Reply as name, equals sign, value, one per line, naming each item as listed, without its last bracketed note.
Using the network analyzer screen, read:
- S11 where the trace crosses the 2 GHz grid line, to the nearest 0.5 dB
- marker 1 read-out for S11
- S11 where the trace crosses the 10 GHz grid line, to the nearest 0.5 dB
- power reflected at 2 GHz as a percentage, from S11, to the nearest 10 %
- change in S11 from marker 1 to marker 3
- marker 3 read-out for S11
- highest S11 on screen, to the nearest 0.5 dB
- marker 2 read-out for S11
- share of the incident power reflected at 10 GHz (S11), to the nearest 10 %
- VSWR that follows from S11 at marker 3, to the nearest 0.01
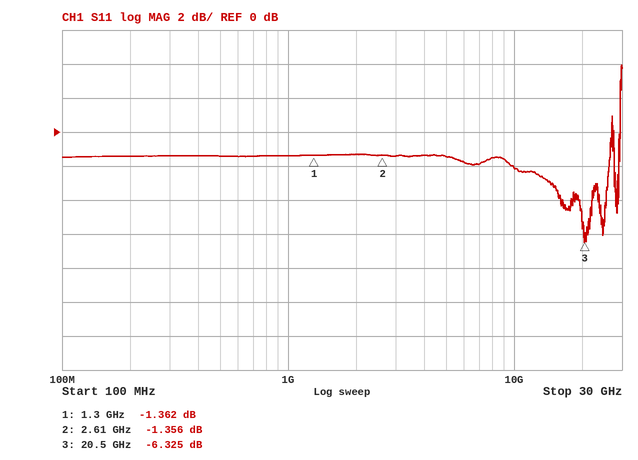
S11 where the trace crosses the 2 GHz grid line, to the nearest 0.5 dB = -1.5 dB
marker 1 read-out for S11 = -1.362 dB
S11 where the trace crosses the 10 GHz grid line, to the nearest 0.5 dB = -2.0 dB
power reflected at 2 GHz as a percentage, from S11, to the nearest 10 % = 70 %
change in S11 from marker 1 to marker 3 = -4.963 dB
marker 3 read-out for S11 = -6.325 dB
highest S11 on screen, to the nearest 0.5 dB = 4.0 dB
marker 2 read-out for S11 = -1.356 dB
share of the incident power reflected at 10 GHz (S11), to the nearest 10 % = 60 %
VSWR that follows from S11 at marker 3, to the nearest 0.01 = 2.87
